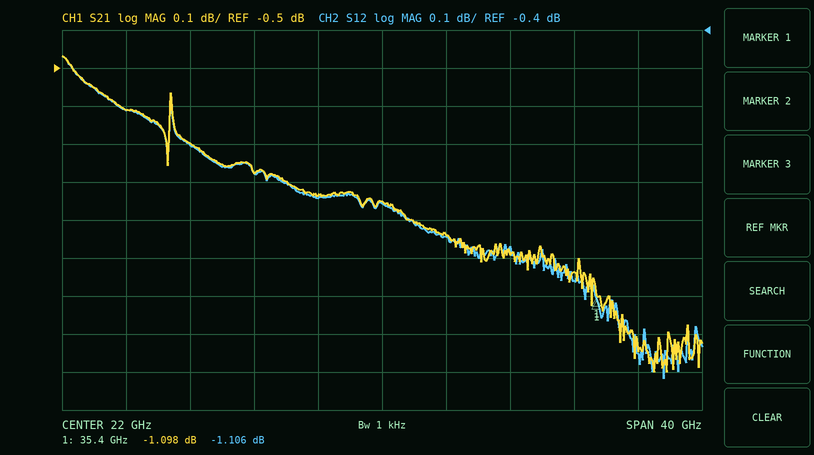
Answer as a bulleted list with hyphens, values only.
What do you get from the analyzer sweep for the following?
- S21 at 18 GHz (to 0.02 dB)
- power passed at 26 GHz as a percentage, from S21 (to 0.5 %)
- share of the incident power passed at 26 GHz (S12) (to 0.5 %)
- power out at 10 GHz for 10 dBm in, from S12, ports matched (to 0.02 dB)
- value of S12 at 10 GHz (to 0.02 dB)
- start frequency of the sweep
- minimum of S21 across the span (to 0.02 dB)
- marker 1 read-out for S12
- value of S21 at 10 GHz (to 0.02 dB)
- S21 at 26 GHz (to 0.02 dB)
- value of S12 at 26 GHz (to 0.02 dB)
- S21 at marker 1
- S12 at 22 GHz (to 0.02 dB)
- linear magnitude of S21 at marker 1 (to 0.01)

- -0.84 dB
- 80.5 %
- 80.5 %
- 9.30 dBm
- -0.70 dB
- 2 GHz
- -1.30 dB
- -1.106 dB
- -0.70 dB
- -0.94 dB
- -0.94 dB
- -1.098 dB
- -0.86 dB
- 0.88
